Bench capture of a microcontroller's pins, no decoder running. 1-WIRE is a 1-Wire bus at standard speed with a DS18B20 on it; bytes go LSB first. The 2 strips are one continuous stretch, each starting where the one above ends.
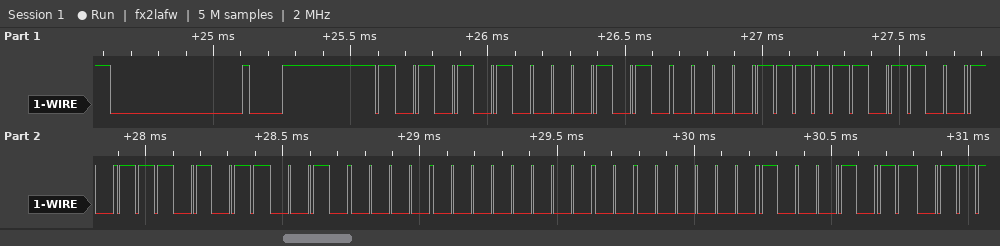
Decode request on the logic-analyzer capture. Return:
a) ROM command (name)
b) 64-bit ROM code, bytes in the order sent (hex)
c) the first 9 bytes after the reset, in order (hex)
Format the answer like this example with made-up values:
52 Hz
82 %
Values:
Match ROM
28 F8 4D D7 04 00 00 D1
55 28 F8 4D D7 04 00 00 D1
